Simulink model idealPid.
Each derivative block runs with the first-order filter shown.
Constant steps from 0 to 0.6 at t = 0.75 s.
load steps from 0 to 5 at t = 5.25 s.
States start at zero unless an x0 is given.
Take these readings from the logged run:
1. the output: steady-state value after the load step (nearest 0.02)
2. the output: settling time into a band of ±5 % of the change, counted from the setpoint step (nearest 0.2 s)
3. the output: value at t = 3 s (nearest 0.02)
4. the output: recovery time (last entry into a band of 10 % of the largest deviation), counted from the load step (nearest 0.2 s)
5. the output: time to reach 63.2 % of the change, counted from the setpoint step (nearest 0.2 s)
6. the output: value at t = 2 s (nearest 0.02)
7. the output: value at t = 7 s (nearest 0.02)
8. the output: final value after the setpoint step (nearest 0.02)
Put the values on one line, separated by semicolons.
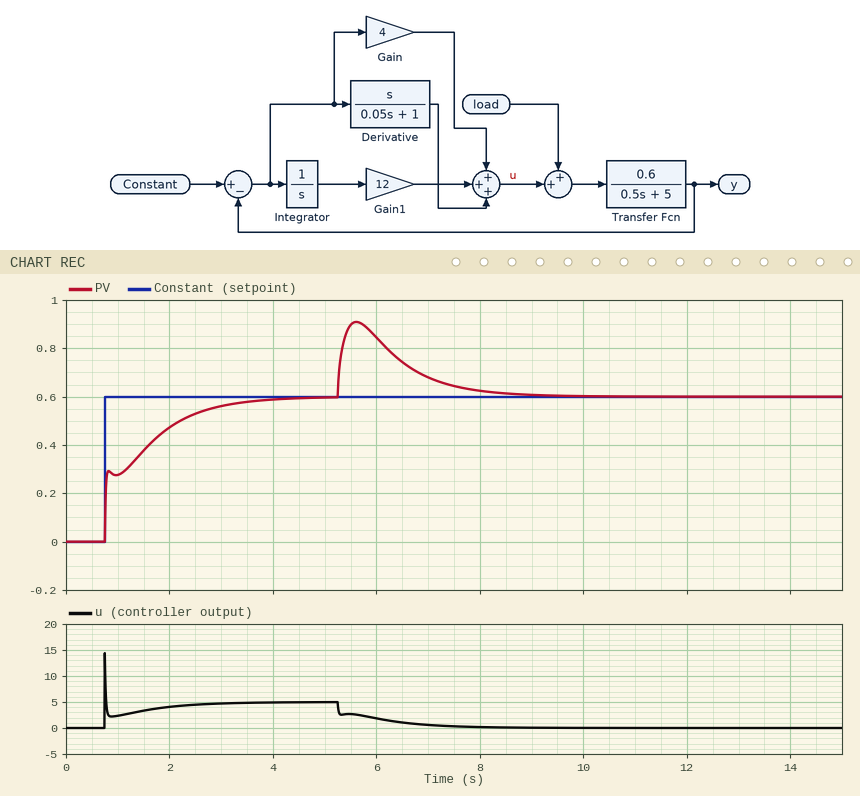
0.60; 2.4 s; 0.56; 2.6 s; 0.8 s; 0.48; 0.68; 0.60
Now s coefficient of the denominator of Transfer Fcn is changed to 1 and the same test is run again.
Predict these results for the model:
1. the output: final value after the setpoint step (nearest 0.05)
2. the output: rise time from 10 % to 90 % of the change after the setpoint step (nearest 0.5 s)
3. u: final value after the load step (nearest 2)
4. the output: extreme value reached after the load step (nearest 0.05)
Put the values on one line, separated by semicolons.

0.60; 2.0 s; 0; 0.90
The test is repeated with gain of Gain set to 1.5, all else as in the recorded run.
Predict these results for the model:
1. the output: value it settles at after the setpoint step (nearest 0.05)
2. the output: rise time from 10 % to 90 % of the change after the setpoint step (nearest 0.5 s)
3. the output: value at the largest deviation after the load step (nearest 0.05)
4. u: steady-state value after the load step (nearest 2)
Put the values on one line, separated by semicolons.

0.60; 1.5 s; 0.95; 0
